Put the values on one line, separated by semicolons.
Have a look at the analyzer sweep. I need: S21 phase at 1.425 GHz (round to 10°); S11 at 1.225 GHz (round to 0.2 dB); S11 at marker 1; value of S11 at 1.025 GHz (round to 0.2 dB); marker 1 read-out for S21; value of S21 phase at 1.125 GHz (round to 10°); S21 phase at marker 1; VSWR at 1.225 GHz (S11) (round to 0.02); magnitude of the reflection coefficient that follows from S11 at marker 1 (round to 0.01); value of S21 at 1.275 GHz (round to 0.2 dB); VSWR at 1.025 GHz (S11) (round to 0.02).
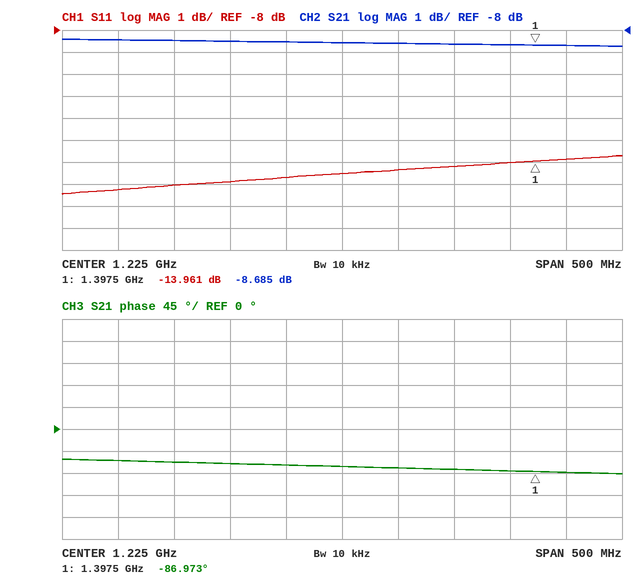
-90°; -14.6 dB; -13.961 dB; -15.2 dB; -8.685 dB; -70°; -86.973°; 1.46; 0.20; -8.6 dB; 1.42
